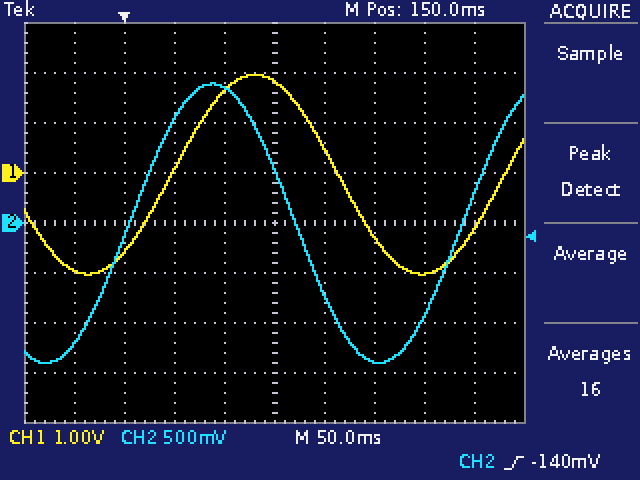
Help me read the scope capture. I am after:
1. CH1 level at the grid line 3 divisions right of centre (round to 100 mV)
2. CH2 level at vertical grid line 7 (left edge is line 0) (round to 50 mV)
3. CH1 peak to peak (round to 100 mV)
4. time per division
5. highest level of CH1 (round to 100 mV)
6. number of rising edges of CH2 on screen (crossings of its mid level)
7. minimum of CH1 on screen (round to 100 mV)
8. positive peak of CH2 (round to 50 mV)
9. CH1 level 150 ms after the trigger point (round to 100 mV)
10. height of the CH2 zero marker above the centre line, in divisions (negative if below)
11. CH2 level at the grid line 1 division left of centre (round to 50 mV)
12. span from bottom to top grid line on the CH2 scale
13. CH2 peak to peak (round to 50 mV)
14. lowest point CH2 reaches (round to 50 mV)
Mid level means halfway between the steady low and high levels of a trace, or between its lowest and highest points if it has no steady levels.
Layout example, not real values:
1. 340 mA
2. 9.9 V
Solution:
1. -2.0 V
2. -1.40 V
3. 4.0 V
4. 50 ms
5. 2.0 V
6. 2
7. -2.0 V
8. 1.40 V
9. 1.8 V
10. 0.0 div
11. 1.35 V
12. 4 V
13. 2.80 V
14. -1.40 V
